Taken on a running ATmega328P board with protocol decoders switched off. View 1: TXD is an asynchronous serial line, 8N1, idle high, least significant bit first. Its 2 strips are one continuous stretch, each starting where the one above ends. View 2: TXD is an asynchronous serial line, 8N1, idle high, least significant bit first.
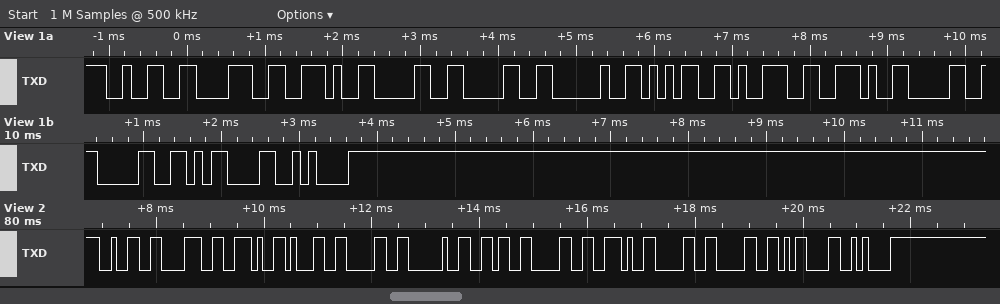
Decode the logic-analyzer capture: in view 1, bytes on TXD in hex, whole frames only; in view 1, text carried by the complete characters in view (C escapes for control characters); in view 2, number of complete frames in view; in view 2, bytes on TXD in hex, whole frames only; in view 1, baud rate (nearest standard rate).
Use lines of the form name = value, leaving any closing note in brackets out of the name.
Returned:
in view 1, bytes on TXD in hex, whole frames only = 0x32 0x38 0x2E 0x30 0x30 0x20 0x35 0x39 0x2E 0x30 0x30 0x0D 0x0A
in view 1, text carried by the complete characters in view = "28.00 59.00\r\n"
in view 2, number of complete frames in view = 13
in view 2, bytes on TXD in hex, whole frames only = 32 38 2E 31 30 20 36 30 2E 30 30 0D 0A
in view 1, baud rate = 9600 baud
